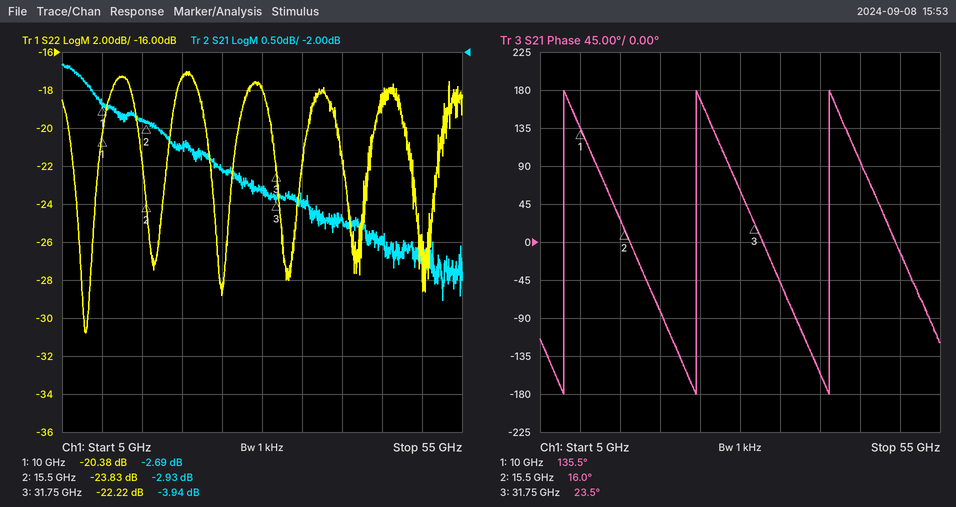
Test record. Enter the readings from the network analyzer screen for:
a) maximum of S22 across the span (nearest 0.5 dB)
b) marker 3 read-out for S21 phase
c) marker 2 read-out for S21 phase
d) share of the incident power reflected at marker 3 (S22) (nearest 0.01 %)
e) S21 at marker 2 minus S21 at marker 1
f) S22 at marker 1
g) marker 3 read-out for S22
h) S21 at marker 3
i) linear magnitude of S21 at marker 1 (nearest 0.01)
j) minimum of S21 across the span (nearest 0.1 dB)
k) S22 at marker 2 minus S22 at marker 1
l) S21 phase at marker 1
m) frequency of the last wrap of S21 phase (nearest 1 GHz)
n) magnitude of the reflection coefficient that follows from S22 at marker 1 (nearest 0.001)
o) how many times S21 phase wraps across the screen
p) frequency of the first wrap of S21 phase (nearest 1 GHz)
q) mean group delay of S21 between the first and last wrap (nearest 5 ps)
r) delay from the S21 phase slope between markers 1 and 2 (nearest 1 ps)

-17.0 dB
23.5°
16.0°
0.60 %
-0.24 dB
-20.38 dB
-22.22 dB
-3.94 dB
0.73
-5.3 dB
-3.45 dB
135.5°
41 GHz
0.096
3
8 GHz
60 ps
60 ps
